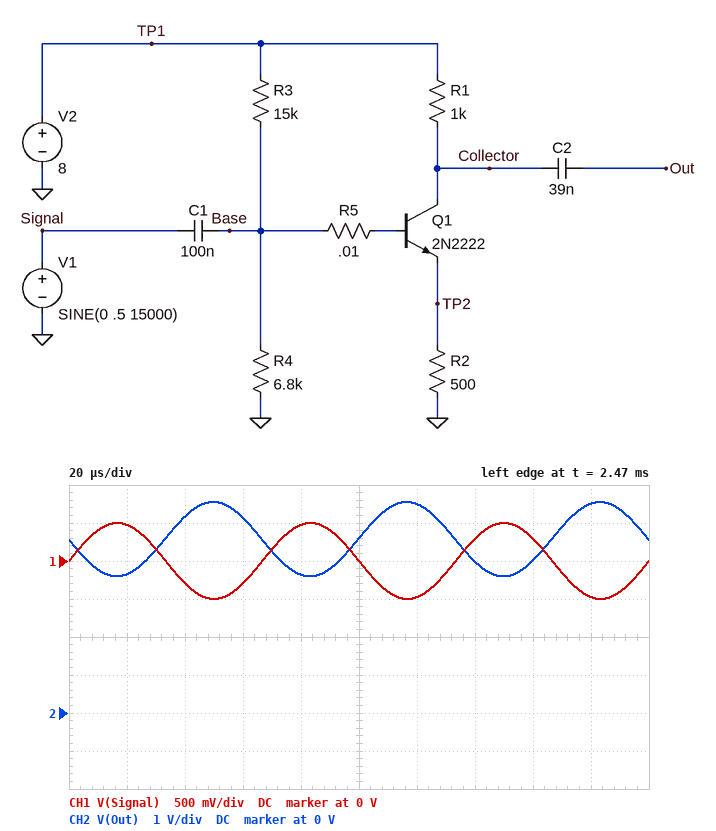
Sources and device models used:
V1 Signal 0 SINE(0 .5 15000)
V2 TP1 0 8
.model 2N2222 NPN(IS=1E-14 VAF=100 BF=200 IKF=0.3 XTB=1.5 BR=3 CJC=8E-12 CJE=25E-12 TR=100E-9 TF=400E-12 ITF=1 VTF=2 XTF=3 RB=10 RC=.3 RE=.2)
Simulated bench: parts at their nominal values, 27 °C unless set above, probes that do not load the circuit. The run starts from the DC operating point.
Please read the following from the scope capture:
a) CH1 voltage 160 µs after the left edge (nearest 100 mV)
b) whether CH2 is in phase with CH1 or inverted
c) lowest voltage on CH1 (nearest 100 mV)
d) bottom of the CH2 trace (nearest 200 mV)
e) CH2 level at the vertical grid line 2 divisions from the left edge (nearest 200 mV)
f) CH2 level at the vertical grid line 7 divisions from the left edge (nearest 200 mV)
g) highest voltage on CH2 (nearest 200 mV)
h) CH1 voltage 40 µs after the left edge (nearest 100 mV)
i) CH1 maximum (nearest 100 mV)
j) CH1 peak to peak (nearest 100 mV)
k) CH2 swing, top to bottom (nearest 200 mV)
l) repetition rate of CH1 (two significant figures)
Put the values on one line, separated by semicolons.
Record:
300 mV; inverted; -500 mV; 3.6 V; 5.2 V; 4.0 V; 5.6 V; -300 mV; 500 mV; 1.0 V; 2.0 V; 15 kHz
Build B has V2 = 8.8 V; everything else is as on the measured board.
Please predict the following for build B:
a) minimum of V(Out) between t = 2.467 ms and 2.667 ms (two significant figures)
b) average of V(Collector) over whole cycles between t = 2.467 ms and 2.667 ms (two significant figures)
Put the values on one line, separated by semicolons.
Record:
3.9 V; 4.9 V
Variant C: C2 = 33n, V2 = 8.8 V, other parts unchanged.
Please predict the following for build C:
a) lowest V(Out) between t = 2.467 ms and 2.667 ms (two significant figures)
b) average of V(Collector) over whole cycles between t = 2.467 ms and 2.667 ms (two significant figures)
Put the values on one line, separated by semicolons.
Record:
3.9 V; 4.9 V
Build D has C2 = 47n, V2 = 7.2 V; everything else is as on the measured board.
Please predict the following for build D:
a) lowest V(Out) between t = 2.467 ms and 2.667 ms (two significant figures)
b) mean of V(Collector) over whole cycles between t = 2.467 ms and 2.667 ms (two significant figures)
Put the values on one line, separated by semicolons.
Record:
3.3 V; 4.2 V
